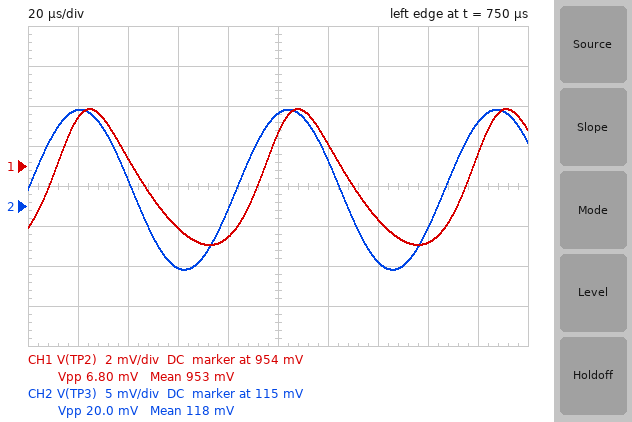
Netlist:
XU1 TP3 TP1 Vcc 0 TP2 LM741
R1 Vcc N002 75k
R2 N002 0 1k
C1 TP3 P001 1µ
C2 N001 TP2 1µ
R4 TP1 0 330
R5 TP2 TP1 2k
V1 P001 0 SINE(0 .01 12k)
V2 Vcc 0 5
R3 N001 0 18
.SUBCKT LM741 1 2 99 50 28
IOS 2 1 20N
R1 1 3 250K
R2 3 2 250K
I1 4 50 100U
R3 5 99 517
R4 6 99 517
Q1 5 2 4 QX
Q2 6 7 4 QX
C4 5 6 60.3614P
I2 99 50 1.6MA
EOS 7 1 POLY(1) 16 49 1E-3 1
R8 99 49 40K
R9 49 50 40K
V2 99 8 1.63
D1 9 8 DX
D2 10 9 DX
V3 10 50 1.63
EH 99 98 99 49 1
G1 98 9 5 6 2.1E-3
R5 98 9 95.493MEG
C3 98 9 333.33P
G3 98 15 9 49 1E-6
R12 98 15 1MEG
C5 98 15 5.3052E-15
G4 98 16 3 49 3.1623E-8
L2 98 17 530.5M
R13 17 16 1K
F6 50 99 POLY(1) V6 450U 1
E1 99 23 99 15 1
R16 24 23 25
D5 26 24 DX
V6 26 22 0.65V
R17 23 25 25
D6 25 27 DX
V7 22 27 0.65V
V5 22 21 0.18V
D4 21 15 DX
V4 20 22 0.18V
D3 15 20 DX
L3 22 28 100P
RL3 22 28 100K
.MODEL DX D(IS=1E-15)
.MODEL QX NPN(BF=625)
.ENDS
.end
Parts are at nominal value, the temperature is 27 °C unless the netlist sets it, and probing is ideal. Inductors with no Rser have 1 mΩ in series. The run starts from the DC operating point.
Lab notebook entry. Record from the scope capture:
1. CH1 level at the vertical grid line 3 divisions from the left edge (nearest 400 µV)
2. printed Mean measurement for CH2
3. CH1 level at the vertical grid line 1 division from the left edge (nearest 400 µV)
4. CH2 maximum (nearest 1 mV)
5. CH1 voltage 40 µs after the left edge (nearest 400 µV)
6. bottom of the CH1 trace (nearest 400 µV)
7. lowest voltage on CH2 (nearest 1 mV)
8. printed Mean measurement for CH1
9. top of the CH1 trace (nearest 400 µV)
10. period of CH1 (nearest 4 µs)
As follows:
950.8 mV
118 mV
956.4 mV
127 mV
954.4 mV
950.0 mV
107 mV
953 mV
956.8 mV
84 µs
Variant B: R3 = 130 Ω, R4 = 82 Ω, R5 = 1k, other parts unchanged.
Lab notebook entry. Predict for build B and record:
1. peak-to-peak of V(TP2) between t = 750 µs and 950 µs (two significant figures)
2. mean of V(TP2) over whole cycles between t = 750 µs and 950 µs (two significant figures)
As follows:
20 mV
920 mV
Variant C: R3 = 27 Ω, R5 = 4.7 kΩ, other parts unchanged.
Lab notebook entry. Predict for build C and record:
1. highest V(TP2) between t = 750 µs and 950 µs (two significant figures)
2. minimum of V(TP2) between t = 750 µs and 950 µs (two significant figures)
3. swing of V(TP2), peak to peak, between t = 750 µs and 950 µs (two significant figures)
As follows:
980 mV
970 mV
6.5 mV
